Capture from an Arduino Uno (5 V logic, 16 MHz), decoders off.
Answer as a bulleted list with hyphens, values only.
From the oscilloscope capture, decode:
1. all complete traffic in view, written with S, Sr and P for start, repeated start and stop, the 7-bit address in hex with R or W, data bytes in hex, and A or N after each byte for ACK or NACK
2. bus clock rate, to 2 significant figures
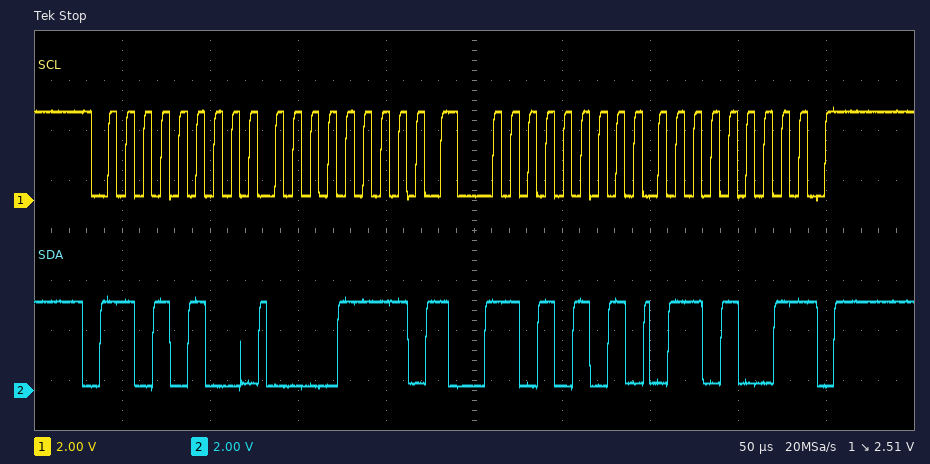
- S 6AW A 0F A Sr 6AR A 69 N P
- 100 kHz
